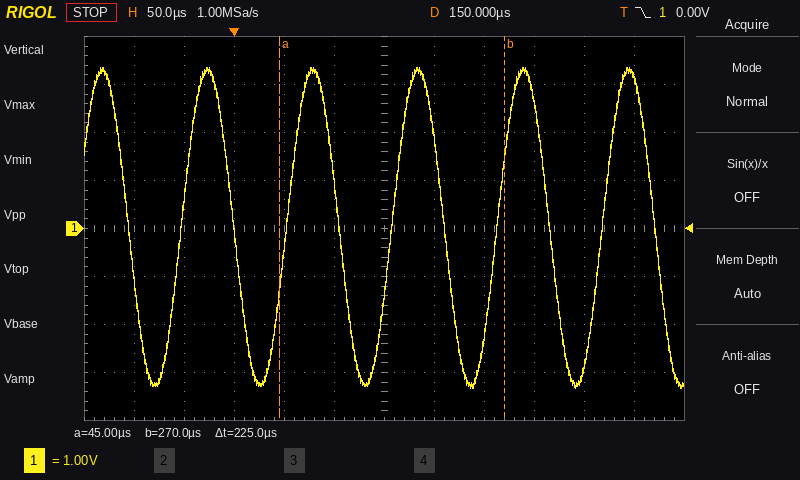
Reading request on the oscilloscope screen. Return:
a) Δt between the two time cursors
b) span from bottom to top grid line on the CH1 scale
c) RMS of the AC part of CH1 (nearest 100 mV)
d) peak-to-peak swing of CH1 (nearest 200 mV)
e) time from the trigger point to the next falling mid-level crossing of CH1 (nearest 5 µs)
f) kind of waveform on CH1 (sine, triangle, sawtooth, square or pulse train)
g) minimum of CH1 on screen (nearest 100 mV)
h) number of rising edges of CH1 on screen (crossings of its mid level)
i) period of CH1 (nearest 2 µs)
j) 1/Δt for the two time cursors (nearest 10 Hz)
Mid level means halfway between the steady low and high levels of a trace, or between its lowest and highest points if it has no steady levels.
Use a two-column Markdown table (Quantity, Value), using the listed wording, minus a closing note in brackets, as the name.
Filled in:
| Quantity | Value |
|---|---|
| Δt between the two time cursors | 225 µs |
| span from bottom to top grid line on the CH1 scale | 8 V |
| RMS of the AC part of CH1 | 2.3 V |
| peak-to-peak swing of CH1 | 6.6 V |
| time from the trigger point to the next falling mid-level crossing of CH1 | 105 µs |
| kind of waveform on CH1 | sine |
| minimum of CH1 on screen | -3.3 V |
| number of rising edges of CH1 on screen | 5 |
| period of CH1 | 106 µs |
| 1/Δt for the two time cursors | 4.44 kHz |
